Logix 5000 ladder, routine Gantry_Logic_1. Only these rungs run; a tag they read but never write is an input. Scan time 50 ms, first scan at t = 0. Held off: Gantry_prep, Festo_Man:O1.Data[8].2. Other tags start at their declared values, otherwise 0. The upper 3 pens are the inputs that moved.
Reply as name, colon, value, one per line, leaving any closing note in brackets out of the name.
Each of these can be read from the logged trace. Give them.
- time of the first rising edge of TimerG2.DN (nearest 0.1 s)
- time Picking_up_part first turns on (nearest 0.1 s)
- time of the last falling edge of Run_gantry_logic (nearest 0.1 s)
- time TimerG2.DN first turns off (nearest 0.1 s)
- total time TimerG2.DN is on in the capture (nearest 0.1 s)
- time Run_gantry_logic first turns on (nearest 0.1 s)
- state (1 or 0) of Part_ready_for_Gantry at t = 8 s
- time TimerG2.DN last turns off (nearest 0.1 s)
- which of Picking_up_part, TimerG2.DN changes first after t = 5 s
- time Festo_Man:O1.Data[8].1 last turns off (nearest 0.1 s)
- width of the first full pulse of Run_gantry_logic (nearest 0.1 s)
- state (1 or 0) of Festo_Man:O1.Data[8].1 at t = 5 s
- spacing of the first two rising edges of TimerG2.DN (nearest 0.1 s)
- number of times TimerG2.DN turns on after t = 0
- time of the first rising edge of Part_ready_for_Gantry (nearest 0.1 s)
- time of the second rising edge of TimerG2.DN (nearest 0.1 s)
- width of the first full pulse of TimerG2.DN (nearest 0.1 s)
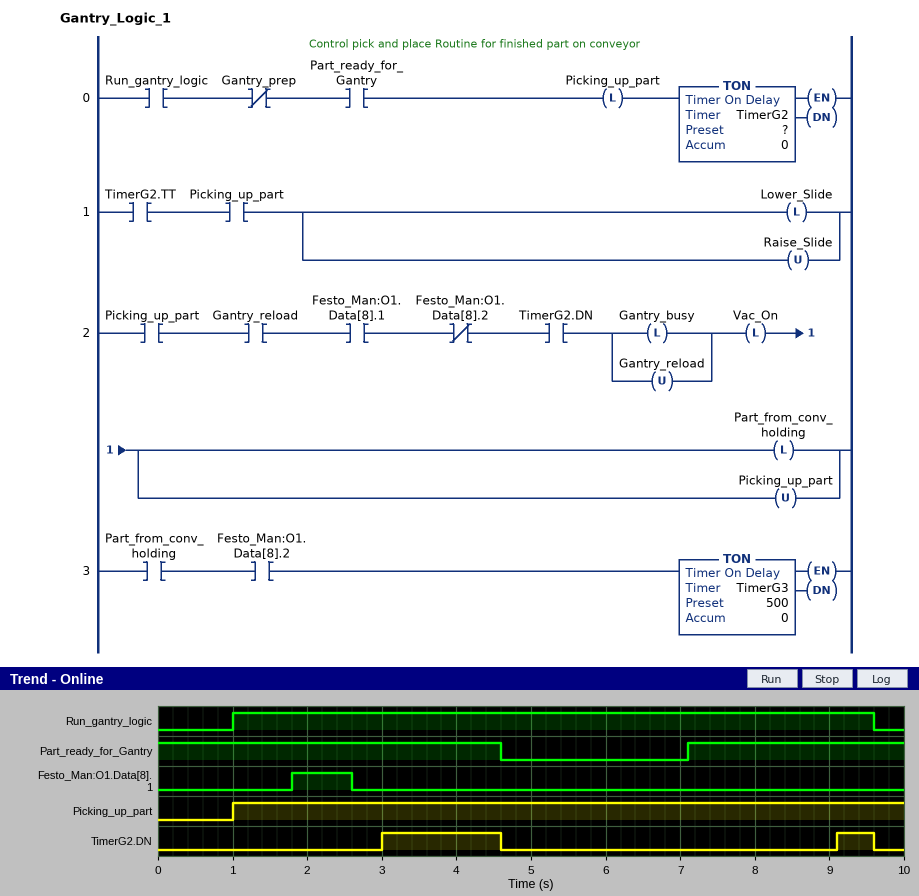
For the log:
time of the first rising edge of TimerG2.DN: 3.0 s
time Picking_up_part first turns on: 1.0 s
time of the last falling edge of Run_gantry_logic: 9.6 s
time TimerG2.DN first turns off: 4.6 s
total time TimerG2.DN is on in the capture: 2.1 s
time Run_gantry_logic first turns on: 1.0 s
state (1 or 0) of Part_ready_for_Gantry at t = 8 s: 1
time TimerG2.DN last turns off: 9.6 s
which of Picking_up_part, TimerG2.DN changes first after t = 5 s: TimerG2.DN
time Festo_Man:O1.Data[8].1 last turns off: 2.6 s
width of the first full pulse of Run_gantry_logic: 8.6 s
state (1 or 0) of Festo_Man:O1.Data[8].1 at t = 5 s: 0
spacing of the first two rising edges of TimerG2.DN: 6.1 s
number of times TimerG2.DN turns on after t = 0: 2
time of the first rising edge of Part_ready_for_Gantry: 7.1 s
time of the second rising edge of TimerG2.DN: 9.1 s
width of the first full pulse of TimerG2.DN: 1.6 s
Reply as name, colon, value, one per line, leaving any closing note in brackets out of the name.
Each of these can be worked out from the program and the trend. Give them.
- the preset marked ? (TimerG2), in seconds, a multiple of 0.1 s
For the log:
the preset marked ? (TimerG2), in seconds, a multiple of 0.1 s: 2.0 s
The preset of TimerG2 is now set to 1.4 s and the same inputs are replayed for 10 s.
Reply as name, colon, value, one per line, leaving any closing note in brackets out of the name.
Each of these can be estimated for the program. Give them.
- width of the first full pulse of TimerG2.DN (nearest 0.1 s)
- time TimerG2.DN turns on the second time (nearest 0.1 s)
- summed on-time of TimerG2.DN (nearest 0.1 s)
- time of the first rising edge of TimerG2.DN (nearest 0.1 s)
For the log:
width of the first full pulse of TimerG2.DN: 2.2 s
time TimerG2.DN turns on the second time: 8.5 s
summed on-time of TimerG2.DN: 3.3 s
time of the first rising edge of TimerG2.DN: 2.4 s
